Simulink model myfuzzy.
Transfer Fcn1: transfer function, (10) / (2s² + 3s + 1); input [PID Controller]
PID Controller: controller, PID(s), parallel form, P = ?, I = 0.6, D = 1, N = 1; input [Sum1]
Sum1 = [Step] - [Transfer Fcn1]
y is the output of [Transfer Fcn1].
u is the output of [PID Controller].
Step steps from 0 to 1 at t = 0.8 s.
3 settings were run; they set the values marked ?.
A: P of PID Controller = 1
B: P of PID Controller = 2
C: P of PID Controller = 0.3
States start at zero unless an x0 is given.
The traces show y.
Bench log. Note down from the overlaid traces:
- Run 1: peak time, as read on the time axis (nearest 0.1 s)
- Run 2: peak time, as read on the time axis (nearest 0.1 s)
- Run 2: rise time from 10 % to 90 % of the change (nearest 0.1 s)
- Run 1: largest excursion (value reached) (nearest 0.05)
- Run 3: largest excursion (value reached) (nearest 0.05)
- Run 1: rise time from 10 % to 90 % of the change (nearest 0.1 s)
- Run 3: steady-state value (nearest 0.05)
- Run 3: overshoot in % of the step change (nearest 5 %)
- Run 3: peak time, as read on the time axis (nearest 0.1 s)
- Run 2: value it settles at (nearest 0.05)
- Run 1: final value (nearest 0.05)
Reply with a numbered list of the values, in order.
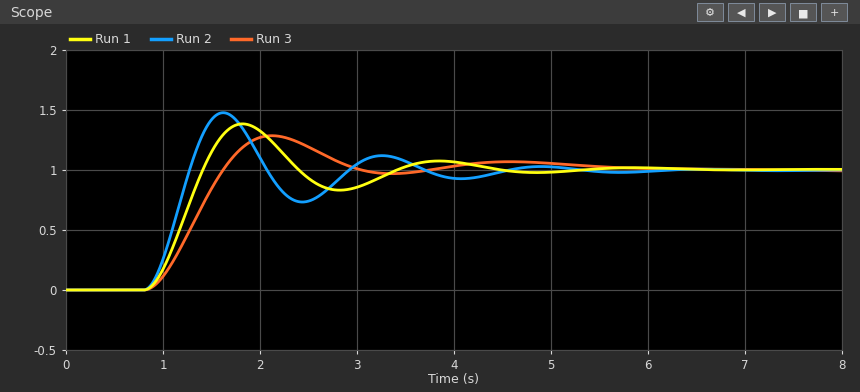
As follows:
1. 1.8 s
2. 1.6 s
3. 0.3 s
4. 1.40
5. 1.30
6. 0.4 s
7. 1.00
8. 30 %
9. 2.1 s
10. 1.00
11. 1.00
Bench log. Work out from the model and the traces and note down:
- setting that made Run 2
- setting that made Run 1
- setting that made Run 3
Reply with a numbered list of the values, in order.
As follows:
1. B
2. A
3. C
